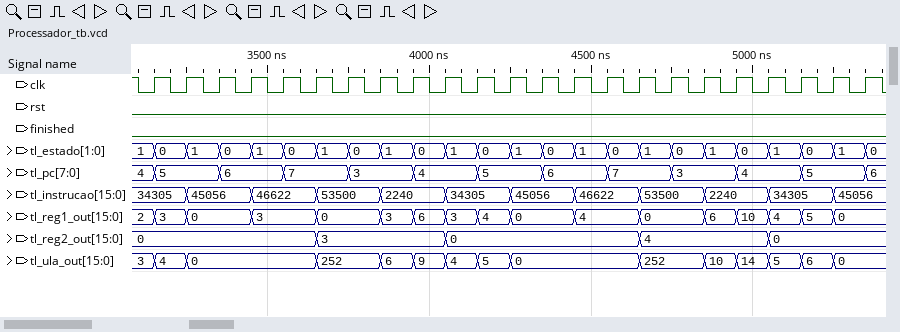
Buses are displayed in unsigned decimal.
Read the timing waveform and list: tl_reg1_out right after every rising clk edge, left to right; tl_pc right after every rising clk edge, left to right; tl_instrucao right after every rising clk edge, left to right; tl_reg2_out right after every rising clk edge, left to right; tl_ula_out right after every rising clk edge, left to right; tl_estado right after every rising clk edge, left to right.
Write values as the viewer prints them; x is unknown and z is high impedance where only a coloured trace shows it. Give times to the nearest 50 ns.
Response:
3, 0, 0, 3, 3, 0, 0, 3, 6, 3, 4, 0, 0, 4, 4, 0, 0, 6, 10, 4, 5, 0, 0
5, 5, 6, 6, 7, 7, 3, 3, 4, 4, 5, 5, 6, 6, 7, 7, 3, 3, 4, 4, 5, 5, 6
34305, 45056, 45056, 46622, 46622, 53500, 53500, 2240, 2240, 34305, 34305, 45056, 45056, 46622, 46622, 53500, 53500, 2240, 2240, 34305, 34305, 45056, 45056
0, 0, 0, 0, 0, 3, 3, 3, 3, 0, 0, 0, 0, 0, 0, 4, 4, 4, 4, 0, 0, 0, 0
4, 0, 0, 0, 0, 252, 252, 6, 9, 4, 5, 0, 0, 0, 0, 252, 252, 10, 14, 5, 6, 0, 0
0, 1, 0, 1, 0, 1, 0, 1, 0, 1, 0, 1, 0, 1, 0, 1, 0, 1, 0, 1, 0, 1, 0
